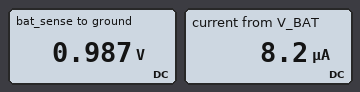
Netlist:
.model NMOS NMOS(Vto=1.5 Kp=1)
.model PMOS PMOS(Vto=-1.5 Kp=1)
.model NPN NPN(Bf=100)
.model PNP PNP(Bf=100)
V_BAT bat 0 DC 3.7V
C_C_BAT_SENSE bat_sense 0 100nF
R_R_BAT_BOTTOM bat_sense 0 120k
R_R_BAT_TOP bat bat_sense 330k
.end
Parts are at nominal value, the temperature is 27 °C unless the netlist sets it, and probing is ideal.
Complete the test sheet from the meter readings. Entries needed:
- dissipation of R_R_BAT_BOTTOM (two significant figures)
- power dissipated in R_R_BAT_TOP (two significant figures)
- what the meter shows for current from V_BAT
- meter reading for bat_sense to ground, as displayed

8.1 µW
22 µW
8.2 µA
0.987 V
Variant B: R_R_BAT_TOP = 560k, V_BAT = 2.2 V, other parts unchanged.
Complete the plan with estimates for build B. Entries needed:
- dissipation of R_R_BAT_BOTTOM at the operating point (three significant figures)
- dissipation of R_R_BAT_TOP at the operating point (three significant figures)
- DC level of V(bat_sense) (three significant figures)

1.26 µW
5.86 µW
388 mV
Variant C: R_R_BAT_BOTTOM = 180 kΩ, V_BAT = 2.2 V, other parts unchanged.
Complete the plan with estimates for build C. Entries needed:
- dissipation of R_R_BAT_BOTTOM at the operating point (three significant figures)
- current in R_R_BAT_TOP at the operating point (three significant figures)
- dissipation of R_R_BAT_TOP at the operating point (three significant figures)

3.35 µW
4.31 µA
6.14 µW
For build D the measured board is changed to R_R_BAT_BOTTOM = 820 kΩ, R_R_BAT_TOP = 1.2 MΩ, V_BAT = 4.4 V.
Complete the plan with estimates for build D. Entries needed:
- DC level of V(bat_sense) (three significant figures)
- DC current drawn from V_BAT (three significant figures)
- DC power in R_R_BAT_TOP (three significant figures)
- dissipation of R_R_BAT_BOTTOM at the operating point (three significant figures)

1.79 V
2.18 µA
5.69 µW
3.89 µW
